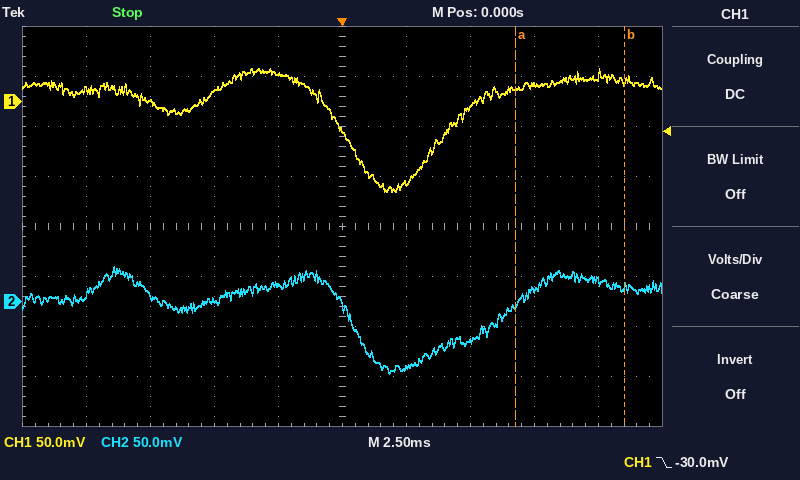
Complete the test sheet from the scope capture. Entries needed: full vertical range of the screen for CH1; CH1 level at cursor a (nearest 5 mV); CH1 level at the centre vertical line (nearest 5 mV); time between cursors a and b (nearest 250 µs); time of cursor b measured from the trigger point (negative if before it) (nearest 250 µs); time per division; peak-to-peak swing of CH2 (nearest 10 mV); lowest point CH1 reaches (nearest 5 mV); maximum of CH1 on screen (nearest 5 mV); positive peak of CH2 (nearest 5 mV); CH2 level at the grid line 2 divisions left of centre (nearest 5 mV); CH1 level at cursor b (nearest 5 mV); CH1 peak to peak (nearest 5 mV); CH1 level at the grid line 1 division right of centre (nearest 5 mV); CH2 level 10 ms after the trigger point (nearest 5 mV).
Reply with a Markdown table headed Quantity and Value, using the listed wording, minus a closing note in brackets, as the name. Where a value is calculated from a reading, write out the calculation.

| Quantity | Value |
|---|---|
| full vertical range of the screen for CH1 | 400 mV |
| CH1 level at cursor a | 15 mV |
| CH1 level at the centre vertical line | -30 mV |
| time between cursors a and b | 4.25 ms |
| time of cursor b measured from the trigger point (negative if before it) | +11.00 ms |
| time per division | 2.5 ms |
| peak-to-peak swing of CH2 | 110 mV |
| lowest point CH1 reaches | -90 mV |
| maximum of CH1 on screen | 35 mV |
| positive peak of CH2 | 35 mV |
| CH2 level at the grid line 2 divisions left of centre | 0 mV |
| CH1 level at cursor b | 20 mV |
| CH1 peak to peak | 35 mV − (-90 mV) = 125 mV |
| CH1 level at the grid line 1 division right of centre | -80 mV |
| CH2 level 10 ms after the trigger point | 20 mV |
